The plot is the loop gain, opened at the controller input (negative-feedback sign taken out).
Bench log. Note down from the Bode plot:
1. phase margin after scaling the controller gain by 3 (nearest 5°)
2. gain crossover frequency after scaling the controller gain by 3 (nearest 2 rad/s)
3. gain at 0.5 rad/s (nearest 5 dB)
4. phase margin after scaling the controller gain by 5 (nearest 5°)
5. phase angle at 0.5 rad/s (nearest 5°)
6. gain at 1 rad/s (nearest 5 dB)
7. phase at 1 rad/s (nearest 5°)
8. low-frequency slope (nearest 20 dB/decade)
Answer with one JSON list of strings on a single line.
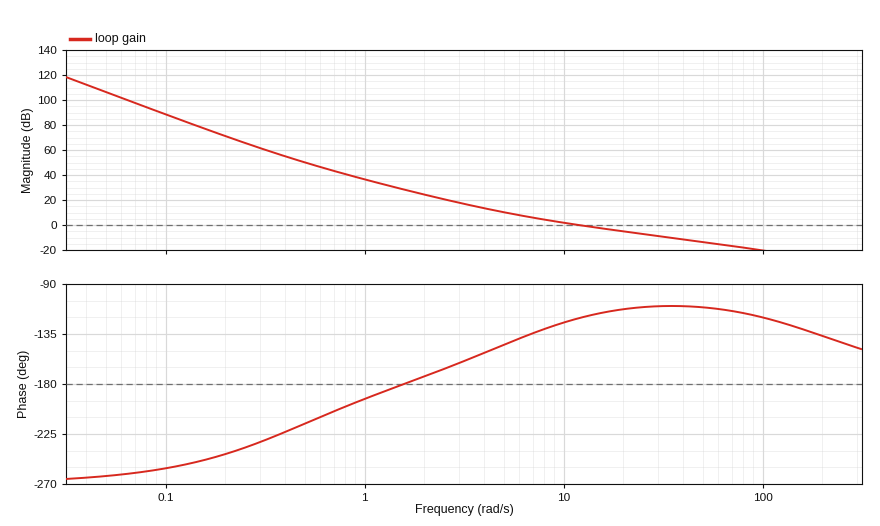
["70°", "32 rad/s", "50 dB", "70°", "-215°", "35 dB", "-195°", "-60 dB/decade"]
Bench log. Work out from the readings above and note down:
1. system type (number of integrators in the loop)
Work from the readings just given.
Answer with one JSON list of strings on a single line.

["3"]
